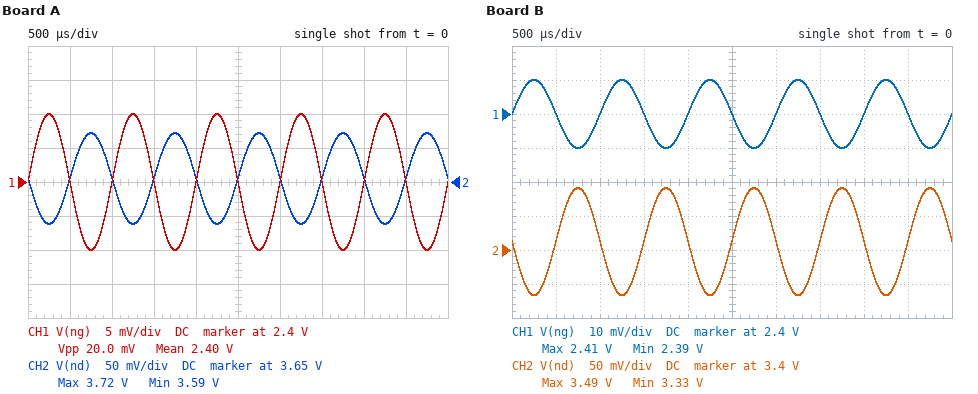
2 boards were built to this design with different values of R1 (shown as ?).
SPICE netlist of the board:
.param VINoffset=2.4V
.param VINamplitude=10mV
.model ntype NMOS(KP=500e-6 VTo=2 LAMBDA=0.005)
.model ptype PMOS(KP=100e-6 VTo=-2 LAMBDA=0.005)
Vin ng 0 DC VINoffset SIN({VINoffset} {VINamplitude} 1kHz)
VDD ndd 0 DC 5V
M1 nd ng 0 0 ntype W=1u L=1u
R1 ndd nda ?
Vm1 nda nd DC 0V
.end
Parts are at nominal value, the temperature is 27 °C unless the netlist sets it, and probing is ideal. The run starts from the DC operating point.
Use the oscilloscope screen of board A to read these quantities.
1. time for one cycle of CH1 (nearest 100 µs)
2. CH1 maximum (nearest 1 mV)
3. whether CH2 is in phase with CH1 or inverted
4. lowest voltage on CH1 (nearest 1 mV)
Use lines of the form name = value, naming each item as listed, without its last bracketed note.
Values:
time for one cycle of CH1 = 1.0 ms
CH1 maximum = 2.410 V
whether CH2 is in phase with CH1 or inverted = inverted
lowest voltage on CH1 = 2.390 V
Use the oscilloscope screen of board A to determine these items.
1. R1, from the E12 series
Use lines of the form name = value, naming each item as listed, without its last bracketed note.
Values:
R1, from the E12 series = 33 kΩ
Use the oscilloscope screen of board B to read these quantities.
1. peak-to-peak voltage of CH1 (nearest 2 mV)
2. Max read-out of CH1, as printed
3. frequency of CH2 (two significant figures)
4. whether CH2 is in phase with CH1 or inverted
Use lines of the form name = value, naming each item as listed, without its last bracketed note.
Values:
peak-to-peak voltage of CH1 = 20 mV
Max read-out of CH1, as printed = 2.41 V
frequency of CH2 = 1.0 kHz
whether CH2 is in phase with CH1 or inverted = inverted
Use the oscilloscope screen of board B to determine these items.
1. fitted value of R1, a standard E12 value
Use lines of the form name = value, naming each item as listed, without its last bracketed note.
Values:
fitted value of R1, a standard E12 value = 39 kΩ
